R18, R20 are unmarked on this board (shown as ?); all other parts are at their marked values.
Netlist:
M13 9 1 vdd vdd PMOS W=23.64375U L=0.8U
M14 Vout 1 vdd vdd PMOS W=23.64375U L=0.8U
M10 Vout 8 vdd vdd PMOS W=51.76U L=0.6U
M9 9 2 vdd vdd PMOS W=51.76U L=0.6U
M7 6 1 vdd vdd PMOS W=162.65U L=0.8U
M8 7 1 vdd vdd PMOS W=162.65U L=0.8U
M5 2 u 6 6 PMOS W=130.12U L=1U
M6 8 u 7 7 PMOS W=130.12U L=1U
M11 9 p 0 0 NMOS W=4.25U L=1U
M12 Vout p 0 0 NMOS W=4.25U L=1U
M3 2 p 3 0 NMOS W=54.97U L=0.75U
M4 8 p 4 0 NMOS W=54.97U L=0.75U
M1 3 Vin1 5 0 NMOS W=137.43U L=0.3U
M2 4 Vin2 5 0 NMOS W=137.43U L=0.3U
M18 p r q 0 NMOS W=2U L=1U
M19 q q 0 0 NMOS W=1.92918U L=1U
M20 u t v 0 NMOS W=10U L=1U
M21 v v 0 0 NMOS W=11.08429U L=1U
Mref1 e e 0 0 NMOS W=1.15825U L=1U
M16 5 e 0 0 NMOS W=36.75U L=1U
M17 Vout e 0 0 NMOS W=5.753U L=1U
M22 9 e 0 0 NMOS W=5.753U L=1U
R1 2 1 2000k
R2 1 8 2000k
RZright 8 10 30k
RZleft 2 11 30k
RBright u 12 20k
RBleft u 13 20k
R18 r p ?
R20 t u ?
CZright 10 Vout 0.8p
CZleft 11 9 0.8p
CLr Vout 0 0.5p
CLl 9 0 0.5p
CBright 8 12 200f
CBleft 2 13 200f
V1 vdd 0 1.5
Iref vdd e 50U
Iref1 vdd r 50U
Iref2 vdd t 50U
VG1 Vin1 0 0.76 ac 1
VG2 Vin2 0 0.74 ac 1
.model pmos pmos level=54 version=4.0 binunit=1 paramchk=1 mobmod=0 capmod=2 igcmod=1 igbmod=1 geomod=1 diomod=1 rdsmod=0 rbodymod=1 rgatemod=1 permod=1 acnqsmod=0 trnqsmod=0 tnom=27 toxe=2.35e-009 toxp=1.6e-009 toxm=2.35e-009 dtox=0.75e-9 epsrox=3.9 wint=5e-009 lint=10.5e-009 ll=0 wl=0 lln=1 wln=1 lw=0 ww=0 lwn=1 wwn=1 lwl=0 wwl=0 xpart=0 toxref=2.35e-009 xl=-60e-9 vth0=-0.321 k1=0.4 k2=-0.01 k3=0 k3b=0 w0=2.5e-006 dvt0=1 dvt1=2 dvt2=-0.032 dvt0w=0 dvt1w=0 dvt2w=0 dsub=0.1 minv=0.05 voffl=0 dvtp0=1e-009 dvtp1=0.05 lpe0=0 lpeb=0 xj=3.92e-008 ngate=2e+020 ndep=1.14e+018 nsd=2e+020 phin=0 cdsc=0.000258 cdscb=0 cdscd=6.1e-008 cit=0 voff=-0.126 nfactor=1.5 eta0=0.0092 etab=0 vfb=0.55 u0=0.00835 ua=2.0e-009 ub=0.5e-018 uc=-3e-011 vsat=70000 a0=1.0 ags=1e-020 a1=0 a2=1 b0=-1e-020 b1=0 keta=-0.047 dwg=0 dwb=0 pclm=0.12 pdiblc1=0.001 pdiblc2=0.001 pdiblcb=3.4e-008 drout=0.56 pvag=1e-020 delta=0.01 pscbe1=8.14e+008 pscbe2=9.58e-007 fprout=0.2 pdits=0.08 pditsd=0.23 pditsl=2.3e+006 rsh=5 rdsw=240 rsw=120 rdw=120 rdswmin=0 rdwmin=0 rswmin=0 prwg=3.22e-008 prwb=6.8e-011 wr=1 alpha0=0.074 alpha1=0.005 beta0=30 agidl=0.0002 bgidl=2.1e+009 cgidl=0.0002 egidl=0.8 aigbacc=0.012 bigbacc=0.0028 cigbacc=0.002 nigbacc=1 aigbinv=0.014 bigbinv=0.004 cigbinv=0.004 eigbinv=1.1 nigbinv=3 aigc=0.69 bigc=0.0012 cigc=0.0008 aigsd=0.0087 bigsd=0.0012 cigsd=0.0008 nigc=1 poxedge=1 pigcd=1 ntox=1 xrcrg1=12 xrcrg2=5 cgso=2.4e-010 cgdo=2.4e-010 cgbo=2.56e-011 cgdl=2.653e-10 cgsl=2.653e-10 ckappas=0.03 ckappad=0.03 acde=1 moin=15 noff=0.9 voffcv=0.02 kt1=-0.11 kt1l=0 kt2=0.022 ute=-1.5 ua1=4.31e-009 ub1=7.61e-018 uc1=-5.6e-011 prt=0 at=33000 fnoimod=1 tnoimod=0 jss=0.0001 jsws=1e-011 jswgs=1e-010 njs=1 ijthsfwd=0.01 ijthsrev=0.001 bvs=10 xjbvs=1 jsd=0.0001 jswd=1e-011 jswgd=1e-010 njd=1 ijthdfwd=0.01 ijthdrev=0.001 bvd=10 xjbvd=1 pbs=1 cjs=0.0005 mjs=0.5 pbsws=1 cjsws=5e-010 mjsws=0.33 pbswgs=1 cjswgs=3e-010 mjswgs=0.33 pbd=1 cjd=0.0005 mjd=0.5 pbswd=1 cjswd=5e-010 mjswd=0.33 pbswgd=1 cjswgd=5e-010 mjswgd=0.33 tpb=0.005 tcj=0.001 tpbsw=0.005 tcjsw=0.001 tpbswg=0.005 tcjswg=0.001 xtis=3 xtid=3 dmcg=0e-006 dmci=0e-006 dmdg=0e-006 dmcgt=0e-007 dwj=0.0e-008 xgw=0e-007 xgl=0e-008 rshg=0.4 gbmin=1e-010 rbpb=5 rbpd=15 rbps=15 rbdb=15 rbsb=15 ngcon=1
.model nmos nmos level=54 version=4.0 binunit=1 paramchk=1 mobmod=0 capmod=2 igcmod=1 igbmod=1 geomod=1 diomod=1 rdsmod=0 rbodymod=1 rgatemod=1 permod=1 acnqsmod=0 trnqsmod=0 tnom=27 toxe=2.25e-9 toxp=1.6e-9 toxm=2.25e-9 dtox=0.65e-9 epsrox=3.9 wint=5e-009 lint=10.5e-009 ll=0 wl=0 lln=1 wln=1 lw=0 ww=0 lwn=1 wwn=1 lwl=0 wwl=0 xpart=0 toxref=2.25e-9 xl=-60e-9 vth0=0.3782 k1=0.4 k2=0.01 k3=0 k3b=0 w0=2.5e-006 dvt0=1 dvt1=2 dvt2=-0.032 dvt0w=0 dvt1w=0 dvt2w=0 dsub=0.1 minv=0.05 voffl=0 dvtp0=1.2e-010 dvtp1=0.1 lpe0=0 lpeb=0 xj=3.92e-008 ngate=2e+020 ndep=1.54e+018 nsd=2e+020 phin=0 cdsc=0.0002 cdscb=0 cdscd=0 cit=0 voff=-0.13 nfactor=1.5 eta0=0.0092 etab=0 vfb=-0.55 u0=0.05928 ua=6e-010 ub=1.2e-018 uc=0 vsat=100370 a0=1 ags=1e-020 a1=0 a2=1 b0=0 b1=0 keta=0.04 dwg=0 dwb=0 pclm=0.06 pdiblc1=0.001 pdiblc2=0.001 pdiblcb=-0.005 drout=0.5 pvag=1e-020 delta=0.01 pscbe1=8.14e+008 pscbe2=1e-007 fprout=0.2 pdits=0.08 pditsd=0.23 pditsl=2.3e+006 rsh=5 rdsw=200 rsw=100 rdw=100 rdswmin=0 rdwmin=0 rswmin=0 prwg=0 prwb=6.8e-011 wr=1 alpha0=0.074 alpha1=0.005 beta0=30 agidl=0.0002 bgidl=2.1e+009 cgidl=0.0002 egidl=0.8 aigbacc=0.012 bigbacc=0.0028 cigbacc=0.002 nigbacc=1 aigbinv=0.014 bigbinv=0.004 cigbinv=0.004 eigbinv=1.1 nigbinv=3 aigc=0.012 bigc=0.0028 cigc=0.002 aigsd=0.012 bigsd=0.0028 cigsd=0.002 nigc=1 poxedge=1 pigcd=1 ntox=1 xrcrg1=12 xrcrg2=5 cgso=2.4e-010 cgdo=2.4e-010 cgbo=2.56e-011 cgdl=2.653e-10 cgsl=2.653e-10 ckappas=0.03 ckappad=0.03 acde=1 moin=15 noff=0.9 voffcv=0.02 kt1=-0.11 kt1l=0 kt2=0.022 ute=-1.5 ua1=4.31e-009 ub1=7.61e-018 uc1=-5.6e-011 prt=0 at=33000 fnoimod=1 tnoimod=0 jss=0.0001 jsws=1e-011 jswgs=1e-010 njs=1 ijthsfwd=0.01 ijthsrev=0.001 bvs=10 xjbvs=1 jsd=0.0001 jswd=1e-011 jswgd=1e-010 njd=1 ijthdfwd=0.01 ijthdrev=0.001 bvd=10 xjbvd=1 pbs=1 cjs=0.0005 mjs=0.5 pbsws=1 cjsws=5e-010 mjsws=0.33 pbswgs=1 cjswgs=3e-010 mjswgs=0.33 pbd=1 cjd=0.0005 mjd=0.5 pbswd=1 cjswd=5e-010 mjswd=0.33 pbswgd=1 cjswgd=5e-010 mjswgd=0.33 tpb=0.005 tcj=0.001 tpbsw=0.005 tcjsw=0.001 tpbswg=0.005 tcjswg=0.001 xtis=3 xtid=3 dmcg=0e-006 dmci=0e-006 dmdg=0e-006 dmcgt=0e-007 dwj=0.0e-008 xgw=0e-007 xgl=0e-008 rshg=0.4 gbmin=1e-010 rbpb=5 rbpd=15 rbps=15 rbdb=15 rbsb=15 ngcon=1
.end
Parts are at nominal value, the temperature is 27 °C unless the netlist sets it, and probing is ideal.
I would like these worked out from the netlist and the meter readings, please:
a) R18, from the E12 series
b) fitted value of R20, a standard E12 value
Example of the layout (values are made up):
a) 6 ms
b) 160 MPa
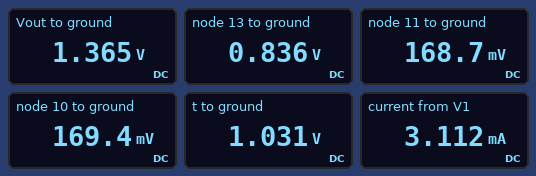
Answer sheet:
a) 3.3 kΩ
b) 3.9 kΩ
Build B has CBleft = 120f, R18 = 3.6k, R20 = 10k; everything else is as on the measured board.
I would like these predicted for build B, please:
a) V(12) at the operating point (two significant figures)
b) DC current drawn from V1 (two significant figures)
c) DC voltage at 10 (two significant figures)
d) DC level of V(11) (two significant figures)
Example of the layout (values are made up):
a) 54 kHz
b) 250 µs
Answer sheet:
a) 550 mV
b) 2.8 mA
c) 1.2 V
d) 460 mV
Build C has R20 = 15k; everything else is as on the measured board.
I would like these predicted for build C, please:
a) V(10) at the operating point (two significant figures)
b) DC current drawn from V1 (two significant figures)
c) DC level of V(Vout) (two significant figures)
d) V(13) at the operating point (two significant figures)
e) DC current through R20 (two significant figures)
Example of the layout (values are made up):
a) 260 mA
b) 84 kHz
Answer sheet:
a) 1.2 V
b) 2.8 mA
c) 44 mV
d) 490 mV
e) 50 µA
